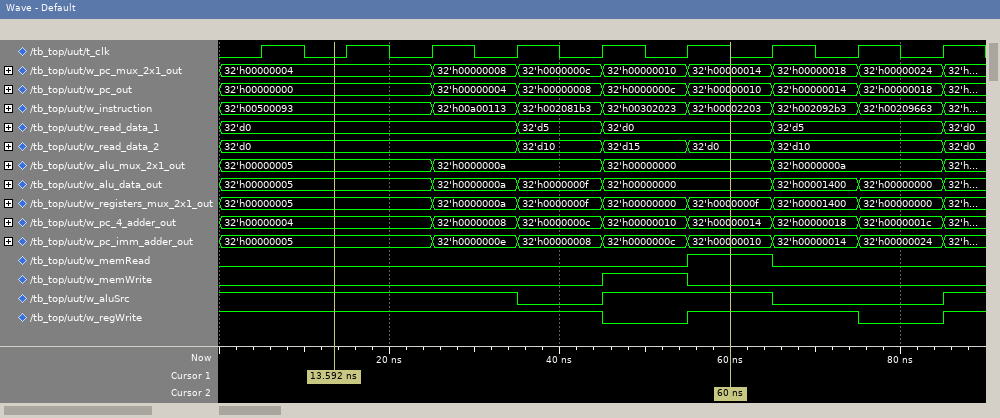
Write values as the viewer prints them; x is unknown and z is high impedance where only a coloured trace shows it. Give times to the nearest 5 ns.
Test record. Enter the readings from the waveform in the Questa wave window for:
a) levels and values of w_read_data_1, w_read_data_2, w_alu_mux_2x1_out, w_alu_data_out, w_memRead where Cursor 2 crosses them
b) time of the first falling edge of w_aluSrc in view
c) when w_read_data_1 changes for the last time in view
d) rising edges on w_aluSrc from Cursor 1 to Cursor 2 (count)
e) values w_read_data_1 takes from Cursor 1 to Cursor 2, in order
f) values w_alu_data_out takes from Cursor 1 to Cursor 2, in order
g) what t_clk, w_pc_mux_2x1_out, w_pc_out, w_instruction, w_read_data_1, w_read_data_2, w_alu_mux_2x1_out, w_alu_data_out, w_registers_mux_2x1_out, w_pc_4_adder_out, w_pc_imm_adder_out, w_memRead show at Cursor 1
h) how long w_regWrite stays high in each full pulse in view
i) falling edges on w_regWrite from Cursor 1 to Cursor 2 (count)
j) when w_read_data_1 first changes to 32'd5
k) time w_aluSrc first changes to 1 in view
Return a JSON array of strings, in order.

["w_read_data_1=32'd0, w_read_data_2=32'd0, w_alu_mux_2x1_out=32'h00000000, w_alu_data_out=32'h00000000, w_memRead=1", "35 ns", "85 ns", "1", "32'd0, 32'd5, 32'd0", "32'h00000005, 32'h0000000a, 32'h0000000f, 32'h00000000", "t_clk=0, w_pc_mux_2x1_out=32'h00000004, w_pc_out=32'h00000000, w_instruction=32'h00500093, w_read_data_1=32'd0, w_read_data_2=32'd0, w_alu_mux_2x1_out=32'h00000005, w_alu_data_out=32'h00000005, w_registers_mux_2x1_out=32'h00000005, w_pc_4_adder_out=32'h00000004, w_pc_imm_adder_out=32'h00000005, w_memRead=0", "20 ns", "1", "35 ns", "45 ns"]
